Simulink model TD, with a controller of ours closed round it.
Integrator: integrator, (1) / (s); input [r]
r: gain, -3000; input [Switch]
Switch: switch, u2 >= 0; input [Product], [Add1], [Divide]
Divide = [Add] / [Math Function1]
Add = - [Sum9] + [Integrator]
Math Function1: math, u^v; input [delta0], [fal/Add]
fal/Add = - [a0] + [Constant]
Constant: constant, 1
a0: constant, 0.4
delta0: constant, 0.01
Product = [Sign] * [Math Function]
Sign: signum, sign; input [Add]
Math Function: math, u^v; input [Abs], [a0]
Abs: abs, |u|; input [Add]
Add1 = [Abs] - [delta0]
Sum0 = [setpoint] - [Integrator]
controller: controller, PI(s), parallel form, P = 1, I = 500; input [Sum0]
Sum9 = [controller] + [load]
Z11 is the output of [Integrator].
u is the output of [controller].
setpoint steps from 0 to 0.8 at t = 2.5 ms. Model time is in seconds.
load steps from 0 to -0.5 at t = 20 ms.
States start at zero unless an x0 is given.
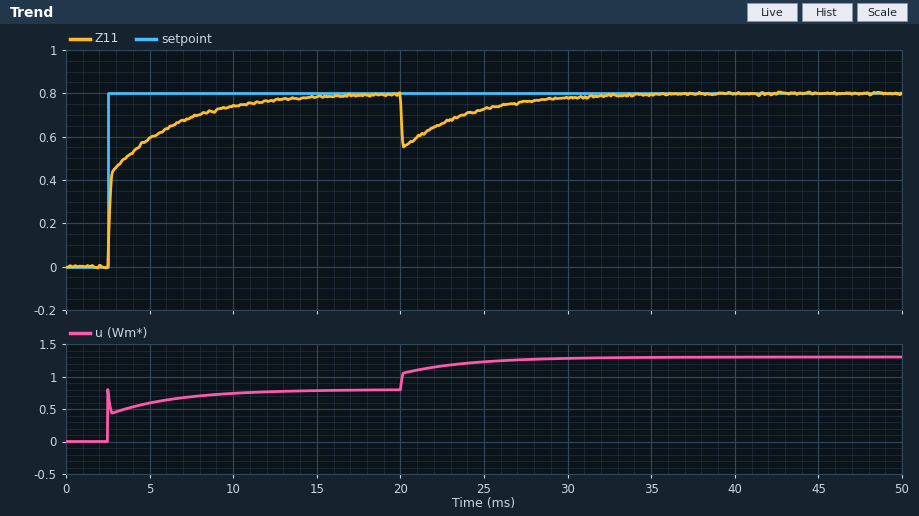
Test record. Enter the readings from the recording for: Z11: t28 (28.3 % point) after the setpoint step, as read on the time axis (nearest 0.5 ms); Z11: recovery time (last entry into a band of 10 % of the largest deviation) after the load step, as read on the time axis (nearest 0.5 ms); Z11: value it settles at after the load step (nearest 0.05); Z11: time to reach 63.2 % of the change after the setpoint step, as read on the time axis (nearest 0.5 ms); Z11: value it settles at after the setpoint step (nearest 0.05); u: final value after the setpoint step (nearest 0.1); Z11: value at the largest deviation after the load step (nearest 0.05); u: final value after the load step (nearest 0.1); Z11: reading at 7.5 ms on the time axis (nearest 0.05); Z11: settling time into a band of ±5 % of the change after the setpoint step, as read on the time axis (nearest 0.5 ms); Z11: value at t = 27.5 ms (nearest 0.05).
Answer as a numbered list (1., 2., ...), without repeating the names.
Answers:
1. 2.5 ms
2. 29.5 ms
3. 0.80
4. 3.5 ms
5. 0.80
6. 0.8
7. 0.55
8. 1.3
9. 0.70
10. 11.5 ms
11. 0.75
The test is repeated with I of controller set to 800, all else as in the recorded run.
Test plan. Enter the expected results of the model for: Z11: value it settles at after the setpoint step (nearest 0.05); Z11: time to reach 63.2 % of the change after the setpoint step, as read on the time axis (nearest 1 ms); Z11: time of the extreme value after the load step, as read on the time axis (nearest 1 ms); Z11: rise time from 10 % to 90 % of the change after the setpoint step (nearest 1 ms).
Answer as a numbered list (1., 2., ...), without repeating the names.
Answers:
1. 0.80
2. 3 ms
3. 20 ms
4. 4 ms
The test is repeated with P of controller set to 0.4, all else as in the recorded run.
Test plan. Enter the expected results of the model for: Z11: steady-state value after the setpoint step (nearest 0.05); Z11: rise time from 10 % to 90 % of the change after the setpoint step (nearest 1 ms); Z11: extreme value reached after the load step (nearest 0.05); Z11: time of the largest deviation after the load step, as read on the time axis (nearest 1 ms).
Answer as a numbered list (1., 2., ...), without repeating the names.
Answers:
1. 0.80
2. 5 ms
3. 0.45
4. 20 ms
